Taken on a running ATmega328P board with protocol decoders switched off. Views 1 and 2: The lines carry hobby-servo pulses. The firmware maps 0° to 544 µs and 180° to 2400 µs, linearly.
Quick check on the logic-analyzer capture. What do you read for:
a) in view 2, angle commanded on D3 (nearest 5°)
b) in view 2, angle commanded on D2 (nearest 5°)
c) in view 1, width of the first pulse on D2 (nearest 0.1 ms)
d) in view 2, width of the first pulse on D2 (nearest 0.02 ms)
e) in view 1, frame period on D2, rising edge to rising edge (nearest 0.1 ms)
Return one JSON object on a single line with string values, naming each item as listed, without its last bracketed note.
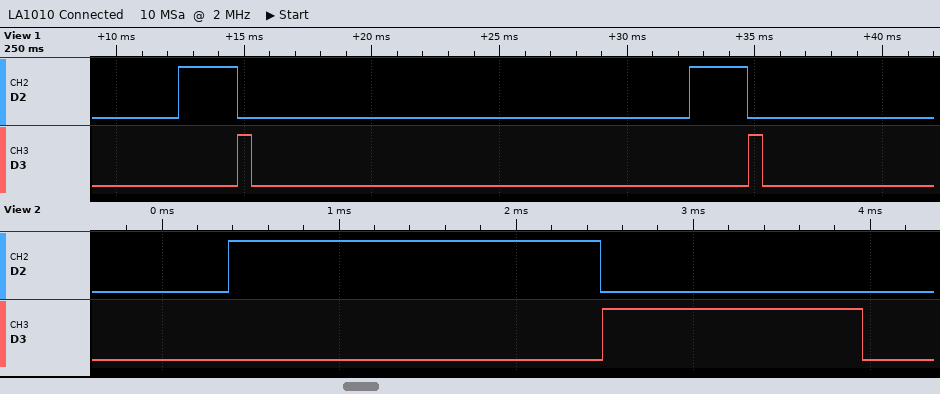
{"in view 2, angle commanded on D3": "90°", "in view 2, angle commanded on D2": "150°", "in view 1, width of the first pulse on D2": "2.3 ms", "in view 2, width of the first pulse on D2": "2.10 ms", "in view 1, frame period on D2, rising edge to rising edge": "20.0 ms"}
